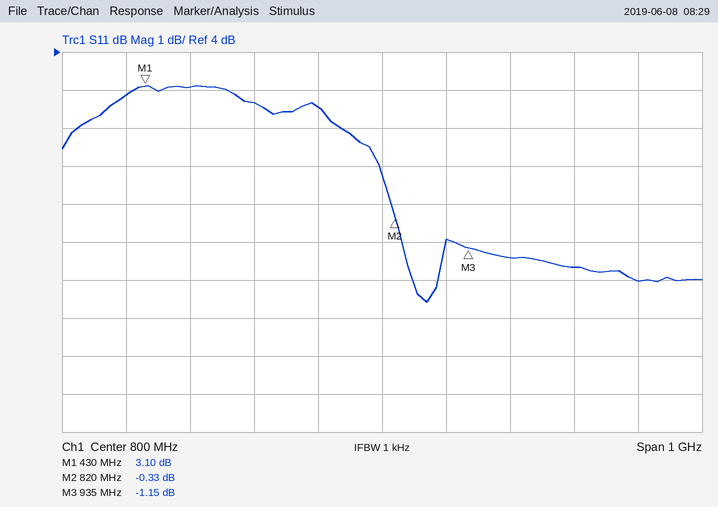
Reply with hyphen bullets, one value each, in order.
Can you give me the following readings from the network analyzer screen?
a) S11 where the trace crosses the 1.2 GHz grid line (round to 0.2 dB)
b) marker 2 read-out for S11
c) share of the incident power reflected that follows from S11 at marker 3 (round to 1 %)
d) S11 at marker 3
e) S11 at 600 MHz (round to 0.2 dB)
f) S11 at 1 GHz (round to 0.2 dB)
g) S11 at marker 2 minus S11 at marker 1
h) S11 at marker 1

- -2.0 dB
- -0.33 dB
- 77 %
- -1.15 dB
- 2.6 dB
- -1.4 dB
- -3.43 dB
- 3.10 dB
